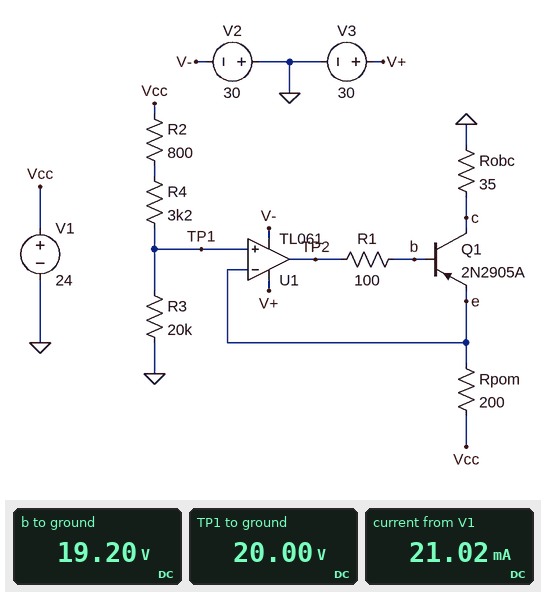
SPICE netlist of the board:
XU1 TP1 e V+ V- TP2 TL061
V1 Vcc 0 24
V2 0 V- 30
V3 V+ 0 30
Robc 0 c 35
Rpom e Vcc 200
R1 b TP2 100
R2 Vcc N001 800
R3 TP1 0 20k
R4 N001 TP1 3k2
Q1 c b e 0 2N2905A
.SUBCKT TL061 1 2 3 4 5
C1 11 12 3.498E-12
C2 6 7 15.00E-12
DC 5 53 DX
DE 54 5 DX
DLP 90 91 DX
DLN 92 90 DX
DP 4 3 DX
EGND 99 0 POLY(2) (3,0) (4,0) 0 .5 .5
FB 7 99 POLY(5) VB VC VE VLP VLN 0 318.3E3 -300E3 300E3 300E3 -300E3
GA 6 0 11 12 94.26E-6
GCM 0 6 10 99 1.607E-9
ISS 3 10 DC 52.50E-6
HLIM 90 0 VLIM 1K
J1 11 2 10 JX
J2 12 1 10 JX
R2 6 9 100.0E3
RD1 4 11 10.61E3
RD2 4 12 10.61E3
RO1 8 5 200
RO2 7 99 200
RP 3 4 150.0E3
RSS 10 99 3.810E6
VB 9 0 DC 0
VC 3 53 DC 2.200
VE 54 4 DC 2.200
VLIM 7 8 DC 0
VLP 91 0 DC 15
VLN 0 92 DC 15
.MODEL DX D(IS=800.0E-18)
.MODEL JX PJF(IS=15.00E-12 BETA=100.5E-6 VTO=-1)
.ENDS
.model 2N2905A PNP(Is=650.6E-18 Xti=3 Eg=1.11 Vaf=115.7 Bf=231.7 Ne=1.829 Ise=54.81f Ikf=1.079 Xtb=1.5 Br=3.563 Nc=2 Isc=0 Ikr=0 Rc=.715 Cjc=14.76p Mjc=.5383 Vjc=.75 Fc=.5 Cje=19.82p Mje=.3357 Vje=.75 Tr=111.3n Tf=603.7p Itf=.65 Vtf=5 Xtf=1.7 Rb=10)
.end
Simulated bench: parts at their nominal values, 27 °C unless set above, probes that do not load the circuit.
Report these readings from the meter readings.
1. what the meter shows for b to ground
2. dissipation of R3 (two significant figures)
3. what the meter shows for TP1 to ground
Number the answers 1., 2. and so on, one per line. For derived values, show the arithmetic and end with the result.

1. 19.20 V
2. (20 V)^2 / 20 kΩ = 20 mW
3. 20.00 V
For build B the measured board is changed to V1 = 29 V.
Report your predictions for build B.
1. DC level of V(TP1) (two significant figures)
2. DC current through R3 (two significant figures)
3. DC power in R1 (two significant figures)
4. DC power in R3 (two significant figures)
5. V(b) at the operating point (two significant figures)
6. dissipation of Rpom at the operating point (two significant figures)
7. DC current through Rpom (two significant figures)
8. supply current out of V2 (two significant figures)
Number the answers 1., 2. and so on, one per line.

1. 24 V
2. 1.2 mA
3. 810 nW
4. 29 mW
5. 23 V
6. 120 mW
7. 24 mA
8. 450 µA
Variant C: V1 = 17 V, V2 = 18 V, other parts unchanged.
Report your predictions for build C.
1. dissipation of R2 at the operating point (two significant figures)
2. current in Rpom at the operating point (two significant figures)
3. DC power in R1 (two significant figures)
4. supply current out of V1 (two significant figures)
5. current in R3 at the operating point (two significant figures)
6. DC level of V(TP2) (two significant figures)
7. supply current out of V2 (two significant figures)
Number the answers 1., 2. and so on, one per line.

1. 400 µW
2. 14 mA
3. 320 nW
4. 15 mA
5. 710 µA
6. 13 V
7. 370 µA
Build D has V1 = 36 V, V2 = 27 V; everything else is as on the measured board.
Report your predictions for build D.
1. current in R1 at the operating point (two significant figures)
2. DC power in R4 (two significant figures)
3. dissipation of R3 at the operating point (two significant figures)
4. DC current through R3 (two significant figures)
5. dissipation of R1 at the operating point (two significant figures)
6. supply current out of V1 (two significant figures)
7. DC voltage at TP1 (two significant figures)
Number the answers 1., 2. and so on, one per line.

1. 120 µA
2. 7.2 mW
3. 45 mW
4. 1.5 mA
5. 1.5 µW
6. 35 mA
7. 30 V
